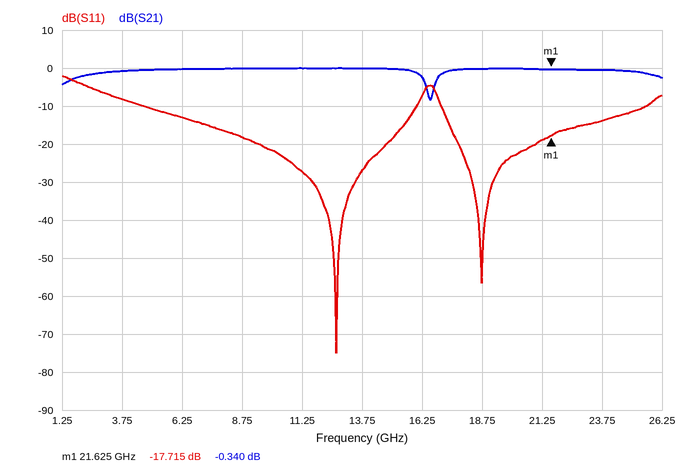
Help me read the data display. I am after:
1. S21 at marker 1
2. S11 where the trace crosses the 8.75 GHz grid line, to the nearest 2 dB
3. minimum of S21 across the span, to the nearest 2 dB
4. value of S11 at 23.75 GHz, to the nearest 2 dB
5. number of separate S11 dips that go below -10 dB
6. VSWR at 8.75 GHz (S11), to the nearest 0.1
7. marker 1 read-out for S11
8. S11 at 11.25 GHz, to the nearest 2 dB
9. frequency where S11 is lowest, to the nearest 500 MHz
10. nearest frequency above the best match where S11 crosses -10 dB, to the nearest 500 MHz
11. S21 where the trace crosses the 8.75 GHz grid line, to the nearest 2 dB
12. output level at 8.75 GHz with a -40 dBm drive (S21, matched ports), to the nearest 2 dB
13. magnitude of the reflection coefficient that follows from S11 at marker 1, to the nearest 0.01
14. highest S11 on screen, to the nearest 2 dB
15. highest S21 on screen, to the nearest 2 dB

-0.340 dB
-18 dB
-8 dB
-14 dB
2
1.3
-17.715 dB
-28 dB
12.5 GHz
16.0 GHz
0 dB
-40 dBm
0.13
-2 dB
0 dB
